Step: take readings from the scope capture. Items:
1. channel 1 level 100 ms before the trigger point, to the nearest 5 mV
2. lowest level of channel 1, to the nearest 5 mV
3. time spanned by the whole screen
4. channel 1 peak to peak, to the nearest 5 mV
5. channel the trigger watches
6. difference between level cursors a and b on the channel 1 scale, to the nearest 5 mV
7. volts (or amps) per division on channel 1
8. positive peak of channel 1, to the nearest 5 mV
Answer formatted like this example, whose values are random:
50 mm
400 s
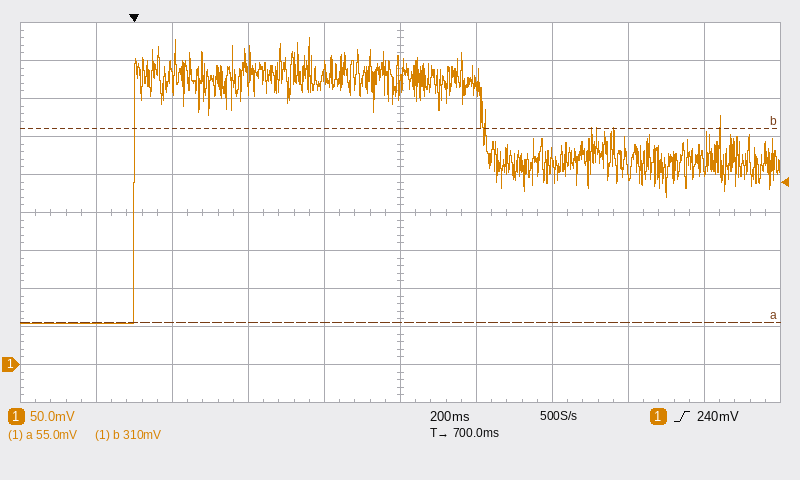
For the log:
55 mV
55 mV
2 s
375 mV
channel 1
255 mV
50 mV
430 mV
